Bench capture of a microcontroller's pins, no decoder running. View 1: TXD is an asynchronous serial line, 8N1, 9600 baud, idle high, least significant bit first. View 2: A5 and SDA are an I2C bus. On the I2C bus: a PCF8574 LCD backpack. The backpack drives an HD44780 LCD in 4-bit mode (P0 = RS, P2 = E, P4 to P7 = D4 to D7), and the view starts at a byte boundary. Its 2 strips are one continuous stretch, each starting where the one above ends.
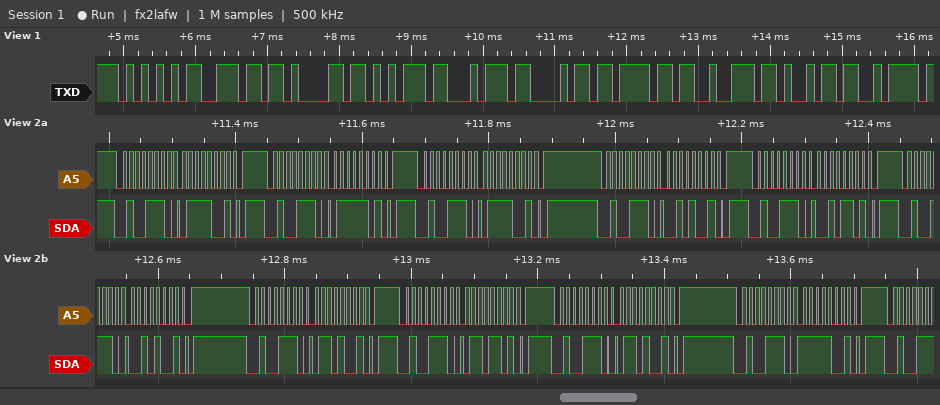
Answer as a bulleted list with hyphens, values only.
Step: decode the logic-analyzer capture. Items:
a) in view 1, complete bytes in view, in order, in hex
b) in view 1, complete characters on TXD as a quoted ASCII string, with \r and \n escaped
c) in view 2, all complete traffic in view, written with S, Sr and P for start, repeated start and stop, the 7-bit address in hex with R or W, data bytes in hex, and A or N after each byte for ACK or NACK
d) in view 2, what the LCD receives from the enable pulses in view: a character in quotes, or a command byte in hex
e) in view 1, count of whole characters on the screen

- 0x55 0x6E 0x61 0x75 0x74 0x68 0x6F 0x72 0x69 0x7A
- "Unauthoriz"
- S 27W A 79 A P S 27W A 7D A P S 27W A 79 A P S 27W A 29 A P S 27W A 2D A P S 27W A 29 A P S 27W A 69 A P S 27W A 6D A P S 27W A 69 A P S 27W A F9 A P
- 'r'
- 10
